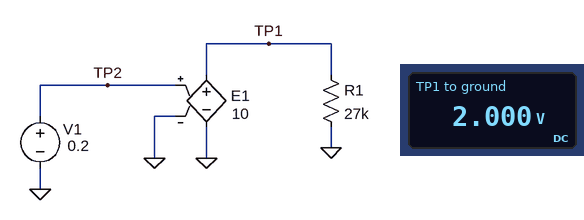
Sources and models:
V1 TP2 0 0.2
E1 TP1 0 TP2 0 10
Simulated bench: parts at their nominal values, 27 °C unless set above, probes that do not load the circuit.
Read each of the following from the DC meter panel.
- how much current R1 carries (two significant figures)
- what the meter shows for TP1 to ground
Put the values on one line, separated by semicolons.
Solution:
74 µA; 2.000 V
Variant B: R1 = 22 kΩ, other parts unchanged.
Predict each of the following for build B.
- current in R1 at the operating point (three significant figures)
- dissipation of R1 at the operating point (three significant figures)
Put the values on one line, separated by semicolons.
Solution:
90.9 µA; 182 µW
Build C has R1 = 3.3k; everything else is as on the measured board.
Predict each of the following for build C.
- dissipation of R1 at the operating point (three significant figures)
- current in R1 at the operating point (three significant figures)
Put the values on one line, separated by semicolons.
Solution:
1.21 mW; 606 µA
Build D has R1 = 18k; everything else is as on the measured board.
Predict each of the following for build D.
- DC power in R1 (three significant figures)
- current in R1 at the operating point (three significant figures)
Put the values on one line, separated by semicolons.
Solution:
222 µW; 111 µA
